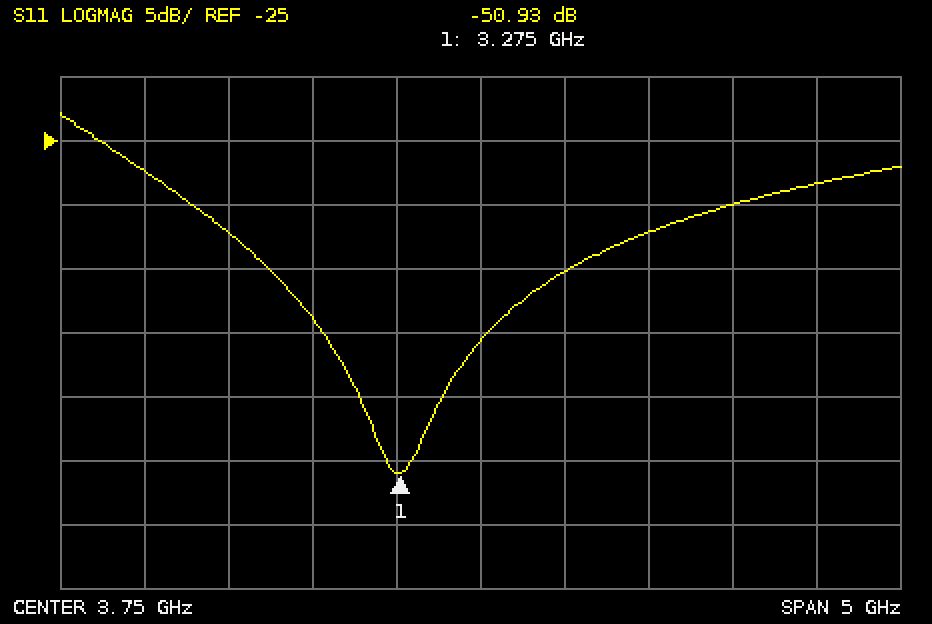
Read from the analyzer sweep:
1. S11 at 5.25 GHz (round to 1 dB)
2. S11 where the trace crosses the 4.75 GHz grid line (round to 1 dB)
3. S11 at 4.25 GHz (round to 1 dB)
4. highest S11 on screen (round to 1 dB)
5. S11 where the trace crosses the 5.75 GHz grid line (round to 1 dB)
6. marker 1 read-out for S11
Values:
-30 dB
-32 dB
-35 dB
-23 dB
-28 dB
-50.93 dB
